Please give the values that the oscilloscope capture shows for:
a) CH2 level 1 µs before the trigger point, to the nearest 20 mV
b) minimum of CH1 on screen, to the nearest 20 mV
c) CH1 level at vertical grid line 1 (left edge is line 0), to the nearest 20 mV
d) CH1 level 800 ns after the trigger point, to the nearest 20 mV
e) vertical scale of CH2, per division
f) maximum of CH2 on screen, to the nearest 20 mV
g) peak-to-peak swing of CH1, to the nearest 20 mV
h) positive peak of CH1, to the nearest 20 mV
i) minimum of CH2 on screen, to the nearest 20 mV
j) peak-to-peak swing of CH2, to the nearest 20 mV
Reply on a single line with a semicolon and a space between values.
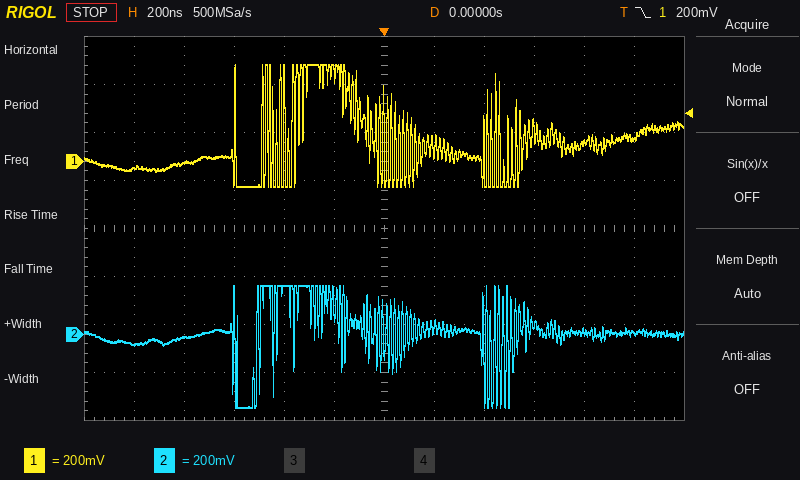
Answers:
-40 mV; -100 mV; -20 mV; 80 mV; 200 mV; 200 mV; 500 mV; 400 mV; -300 mV; 500 mV
